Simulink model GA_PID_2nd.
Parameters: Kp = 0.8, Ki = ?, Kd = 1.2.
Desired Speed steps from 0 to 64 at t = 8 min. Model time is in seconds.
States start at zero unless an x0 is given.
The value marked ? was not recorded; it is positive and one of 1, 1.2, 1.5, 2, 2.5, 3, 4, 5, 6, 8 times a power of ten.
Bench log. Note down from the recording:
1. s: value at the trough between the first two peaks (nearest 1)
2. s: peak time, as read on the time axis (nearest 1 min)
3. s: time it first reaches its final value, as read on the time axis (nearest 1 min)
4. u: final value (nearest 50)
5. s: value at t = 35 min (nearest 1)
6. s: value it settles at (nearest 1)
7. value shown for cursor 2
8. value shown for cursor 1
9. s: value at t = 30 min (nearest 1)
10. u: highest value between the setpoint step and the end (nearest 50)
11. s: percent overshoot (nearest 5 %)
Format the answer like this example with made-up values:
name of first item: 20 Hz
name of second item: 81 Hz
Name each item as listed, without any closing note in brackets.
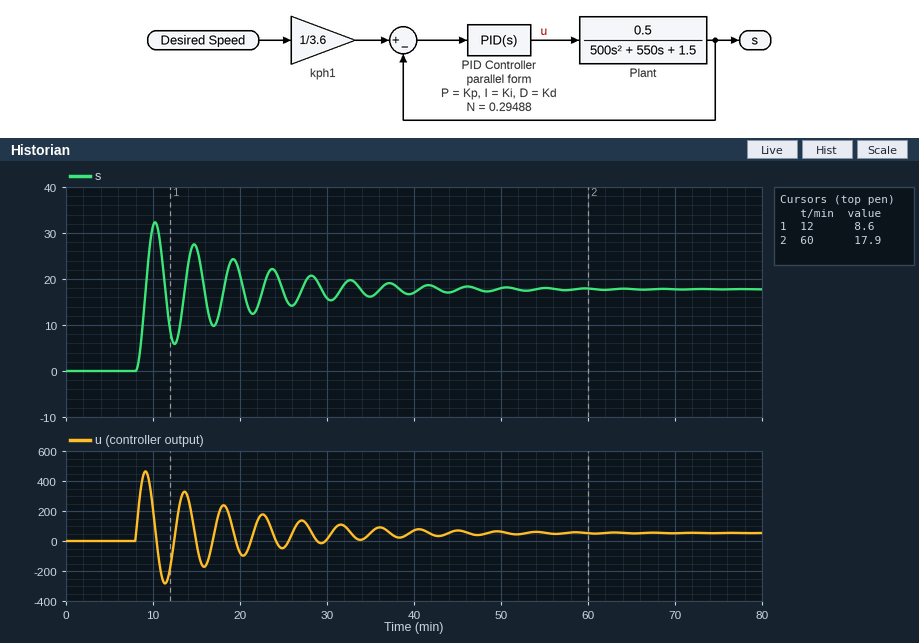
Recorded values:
s: value at the trough between the first two peaks: 6
s: peak time, as read on the time axis: 10 min
s: time it first reaches its final value, as read on the time axis: 9 min
u: final value: 50
s: value at t = 35 min: 16
s: value it settles at: 18
value shown for cursor 2: 17.9
value shown for cursor 1: 8.6
s: value at t = 30 min: 16
u: highest value between the setpoint step and the end: 450
s: percent overshoot: 80 %
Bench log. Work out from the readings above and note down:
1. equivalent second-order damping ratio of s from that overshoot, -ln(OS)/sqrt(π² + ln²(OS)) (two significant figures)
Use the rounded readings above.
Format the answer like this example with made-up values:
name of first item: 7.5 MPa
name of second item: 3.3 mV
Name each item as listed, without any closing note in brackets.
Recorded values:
equivalent second-order damping ratio of s from that overshoot, -ln(OS)/sqrt(π² + ln²(OS)): 0.071
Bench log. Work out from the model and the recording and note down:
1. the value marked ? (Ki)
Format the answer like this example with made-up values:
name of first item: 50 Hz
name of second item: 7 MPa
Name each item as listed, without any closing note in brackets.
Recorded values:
the value marked ?: 0.6
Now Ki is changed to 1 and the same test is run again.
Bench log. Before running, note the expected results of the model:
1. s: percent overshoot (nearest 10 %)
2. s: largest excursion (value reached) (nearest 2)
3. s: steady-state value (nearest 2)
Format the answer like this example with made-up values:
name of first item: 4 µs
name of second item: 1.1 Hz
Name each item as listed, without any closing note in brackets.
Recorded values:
s: percent overshoot: 90 %
s: largest excursion (value reached): 34
s: steady-state value: 18
